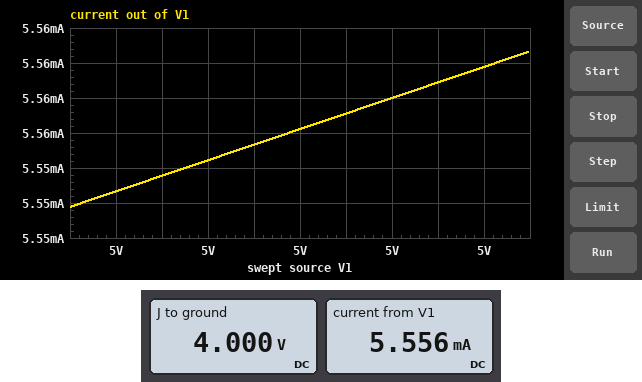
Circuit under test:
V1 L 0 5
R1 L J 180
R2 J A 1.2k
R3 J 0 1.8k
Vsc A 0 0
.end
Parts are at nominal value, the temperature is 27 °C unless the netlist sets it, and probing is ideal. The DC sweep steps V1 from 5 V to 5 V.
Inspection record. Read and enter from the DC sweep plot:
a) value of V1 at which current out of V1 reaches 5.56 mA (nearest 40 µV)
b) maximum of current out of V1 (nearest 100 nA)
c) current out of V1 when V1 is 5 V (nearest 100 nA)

5.00040 V
5.5567 mA
5.5547 mA
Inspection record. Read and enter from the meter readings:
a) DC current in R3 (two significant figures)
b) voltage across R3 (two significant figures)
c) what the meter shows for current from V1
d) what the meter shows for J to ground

2.2 mA
4.0 V
5.556 mA
4.000 V
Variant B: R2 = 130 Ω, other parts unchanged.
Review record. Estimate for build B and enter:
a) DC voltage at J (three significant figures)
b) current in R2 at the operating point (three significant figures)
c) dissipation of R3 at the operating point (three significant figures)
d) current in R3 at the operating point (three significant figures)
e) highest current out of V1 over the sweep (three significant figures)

2.01 V
15.5 mA
2.25 mW
1.12 mA
16.6 mA
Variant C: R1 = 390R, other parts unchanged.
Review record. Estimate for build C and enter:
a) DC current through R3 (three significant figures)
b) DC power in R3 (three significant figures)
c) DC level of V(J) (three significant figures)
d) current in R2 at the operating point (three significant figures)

1.80 mA
5.84 mW
3.24 V
2.70 mA
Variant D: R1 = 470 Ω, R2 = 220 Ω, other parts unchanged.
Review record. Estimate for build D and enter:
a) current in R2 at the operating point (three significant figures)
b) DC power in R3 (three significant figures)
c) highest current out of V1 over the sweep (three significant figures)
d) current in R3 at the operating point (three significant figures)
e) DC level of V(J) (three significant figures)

6.69 mA
1.20 mW
7.51 mA
818 µA
1.47 V
